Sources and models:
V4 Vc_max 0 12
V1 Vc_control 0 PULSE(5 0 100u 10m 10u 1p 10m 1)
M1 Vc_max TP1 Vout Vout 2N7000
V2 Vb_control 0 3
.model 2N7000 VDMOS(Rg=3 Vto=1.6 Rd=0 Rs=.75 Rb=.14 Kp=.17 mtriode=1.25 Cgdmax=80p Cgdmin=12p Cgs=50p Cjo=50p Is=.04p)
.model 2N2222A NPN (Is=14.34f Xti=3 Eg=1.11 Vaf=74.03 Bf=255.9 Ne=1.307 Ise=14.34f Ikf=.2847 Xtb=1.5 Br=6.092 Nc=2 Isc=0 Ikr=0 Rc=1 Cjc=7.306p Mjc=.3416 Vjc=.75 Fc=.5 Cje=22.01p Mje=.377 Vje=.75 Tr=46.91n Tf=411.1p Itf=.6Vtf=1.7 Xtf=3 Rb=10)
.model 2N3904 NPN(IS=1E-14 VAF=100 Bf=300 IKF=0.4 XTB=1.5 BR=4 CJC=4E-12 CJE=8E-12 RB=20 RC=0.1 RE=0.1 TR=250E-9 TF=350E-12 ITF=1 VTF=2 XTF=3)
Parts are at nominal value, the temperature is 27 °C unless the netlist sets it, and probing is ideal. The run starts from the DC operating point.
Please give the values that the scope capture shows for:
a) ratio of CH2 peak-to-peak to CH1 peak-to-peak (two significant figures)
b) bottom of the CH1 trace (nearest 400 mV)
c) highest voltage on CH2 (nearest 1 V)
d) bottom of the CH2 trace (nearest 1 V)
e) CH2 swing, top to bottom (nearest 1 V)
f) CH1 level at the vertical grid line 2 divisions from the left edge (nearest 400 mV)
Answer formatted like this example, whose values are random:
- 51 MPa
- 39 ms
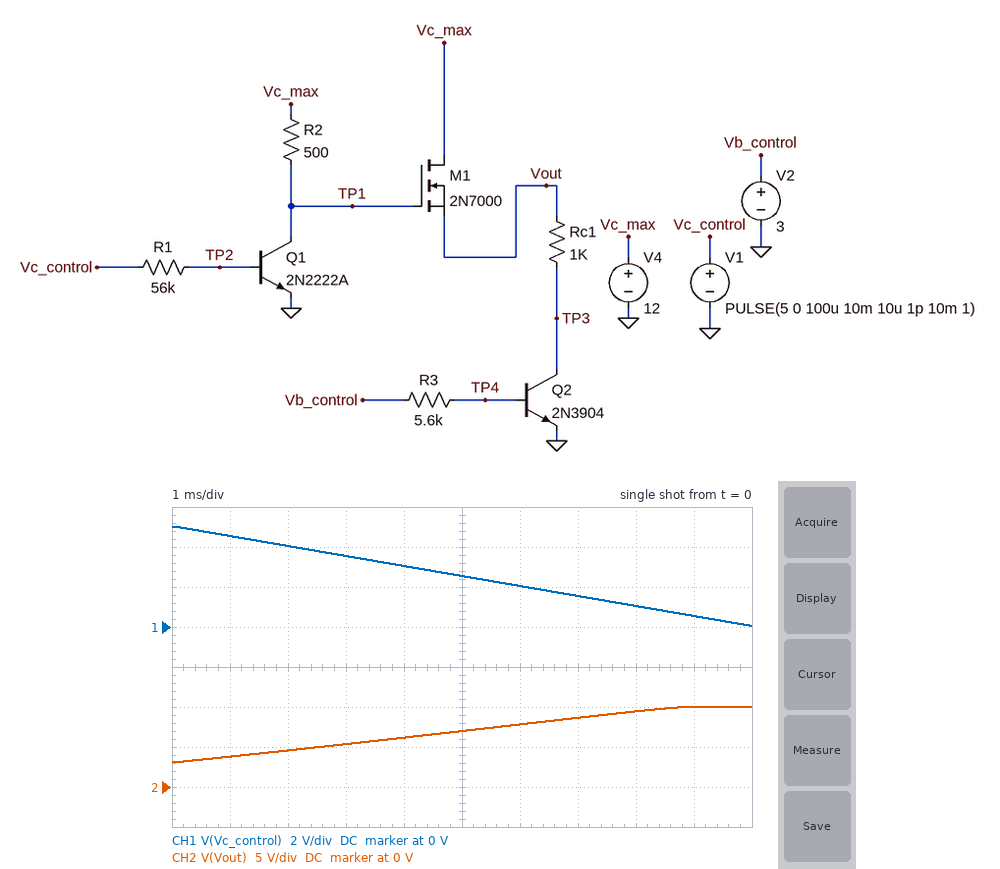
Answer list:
- 1.4
- 0 V
- 10 V
- 3 V
- 7 V
- 4.0 V
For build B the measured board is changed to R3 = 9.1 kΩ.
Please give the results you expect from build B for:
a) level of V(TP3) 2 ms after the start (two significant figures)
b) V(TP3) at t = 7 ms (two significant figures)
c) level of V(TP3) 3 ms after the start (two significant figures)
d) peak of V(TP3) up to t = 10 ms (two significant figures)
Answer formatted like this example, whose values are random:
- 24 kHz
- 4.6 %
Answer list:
- 48 mV
- 65 mV
- 52 mV
- 69 mV
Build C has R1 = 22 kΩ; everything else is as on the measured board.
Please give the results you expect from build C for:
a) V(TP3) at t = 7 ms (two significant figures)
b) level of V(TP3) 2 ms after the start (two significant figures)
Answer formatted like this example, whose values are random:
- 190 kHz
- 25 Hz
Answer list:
- 46 mV
- 5.9 mV
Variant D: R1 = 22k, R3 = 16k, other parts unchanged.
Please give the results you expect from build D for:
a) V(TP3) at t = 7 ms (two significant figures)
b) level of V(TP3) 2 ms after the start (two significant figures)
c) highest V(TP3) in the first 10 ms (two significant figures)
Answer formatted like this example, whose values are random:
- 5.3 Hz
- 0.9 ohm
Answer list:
- 71 mV
- 5.8 mV
- 86 mV
